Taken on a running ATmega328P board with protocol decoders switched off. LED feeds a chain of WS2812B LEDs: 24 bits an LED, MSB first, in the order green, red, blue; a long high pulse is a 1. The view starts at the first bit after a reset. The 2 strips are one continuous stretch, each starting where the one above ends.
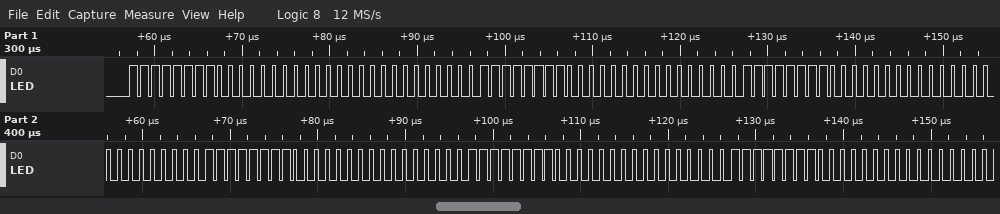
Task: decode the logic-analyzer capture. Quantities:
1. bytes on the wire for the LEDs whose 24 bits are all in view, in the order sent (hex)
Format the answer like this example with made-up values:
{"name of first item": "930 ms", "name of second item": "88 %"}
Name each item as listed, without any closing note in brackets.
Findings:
{"bytes on the wire for the LEDs whose 24 bits are all in view, in the order sent": "FF 00 00 00 FF 00 00 FF 00 00 00 FF 00 00 FF 00 00 FF"}
